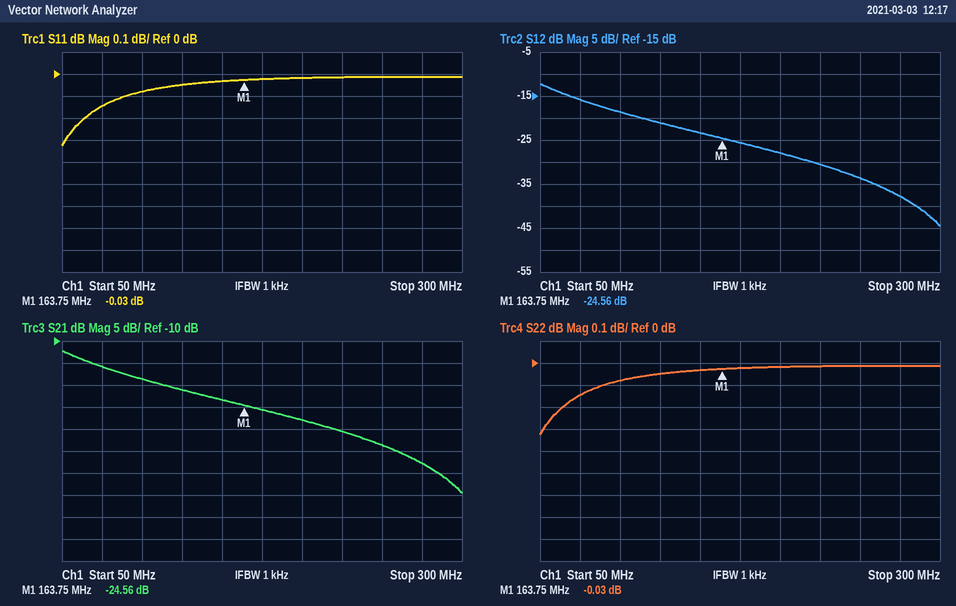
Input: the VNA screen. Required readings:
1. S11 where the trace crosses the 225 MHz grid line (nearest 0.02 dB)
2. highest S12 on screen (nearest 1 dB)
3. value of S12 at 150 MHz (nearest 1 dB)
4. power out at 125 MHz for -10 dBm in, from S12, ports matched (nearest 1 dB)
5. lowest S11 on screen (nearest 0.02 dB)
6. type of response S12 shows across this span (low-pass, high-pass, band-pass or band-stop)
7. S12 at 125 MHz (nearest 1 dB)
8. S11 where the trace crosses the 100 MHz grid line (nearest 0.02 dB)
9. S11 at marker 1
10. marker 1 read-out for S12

-0.02 dB
-12 dB
-23 dB
-31 dBm
-0.32 dB
low-pass
-21 dB
-0.08 dB
-0.03 dB
-24.56 dB
